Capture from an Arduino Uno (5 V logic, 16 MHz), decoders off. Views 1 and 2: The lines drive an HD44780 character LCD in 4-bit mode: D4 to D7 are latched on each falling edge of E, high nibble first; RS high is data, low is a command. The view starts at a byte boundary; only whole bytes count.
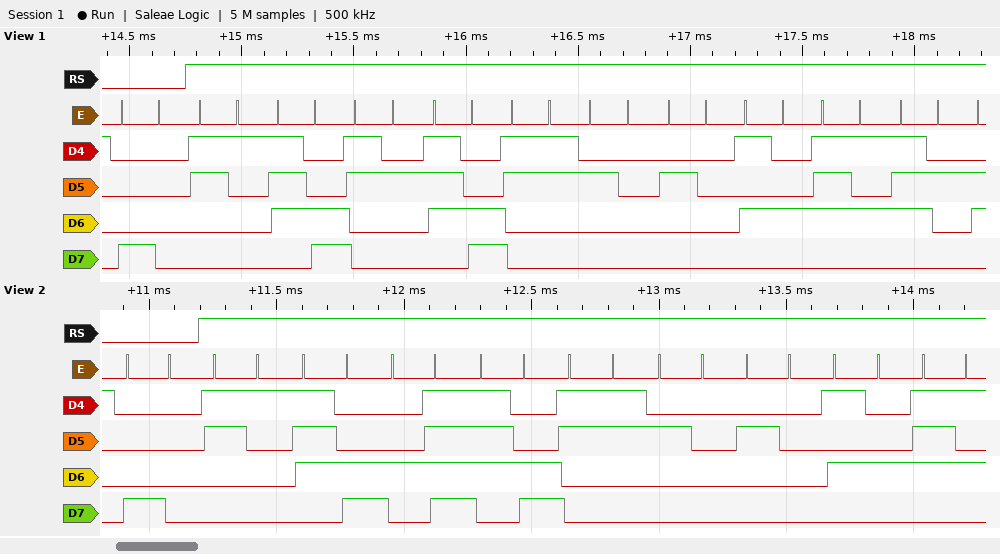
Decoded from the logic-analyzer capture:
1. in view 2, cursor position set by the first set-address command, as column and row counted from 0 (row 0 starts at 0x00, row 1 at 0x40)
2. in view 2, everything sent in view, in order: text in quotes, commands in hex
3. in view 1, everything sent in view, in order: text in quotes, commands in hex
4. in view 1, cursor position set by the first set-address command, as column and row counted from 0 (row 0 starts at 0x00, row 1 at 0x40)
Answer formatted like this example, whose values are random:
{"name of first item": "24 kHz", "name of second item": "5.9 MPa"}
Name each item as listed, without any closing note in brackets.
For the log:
{"in view 2, cursor position set by the first set-address command, as column and row counted from 0": "column 0, row 0", "in view 2, everything sent in view, in order: text in quotes, commands in hex": "0x80 \"1|O|3  Tu\"", "in view 1, everything sent in view, in order: text in quotes, commands in hex": "0x80 \"1|2|3  Tur\"", "in view 1, cursor position set by the first set-address command, as column and row counted from 0": "column 0, row 0"}
